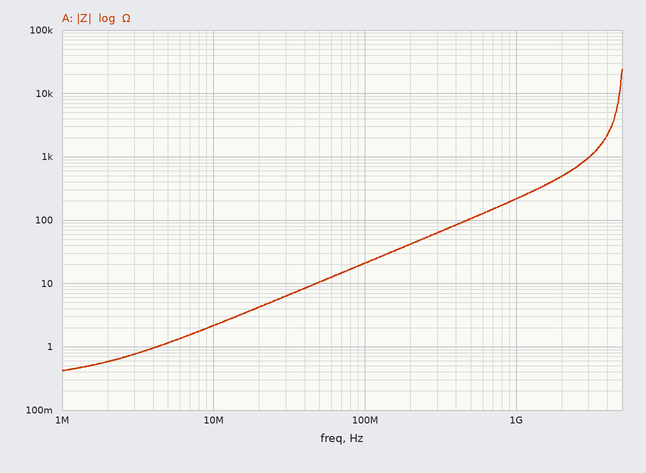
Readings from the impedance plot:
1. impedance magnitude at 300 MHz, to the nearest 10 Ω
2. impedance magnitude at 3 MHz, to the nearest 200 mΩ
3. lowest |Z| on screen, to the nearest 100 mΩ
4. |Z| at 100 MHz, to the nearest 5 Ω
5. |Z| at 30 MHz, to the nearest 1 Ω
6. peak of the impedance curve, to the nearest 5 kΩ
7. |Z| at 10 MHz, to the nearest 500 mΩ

60 Ω
800 mΩ
400 mΩ
20 Ω
6 Ω
25 kΩ
2.0 Ω
